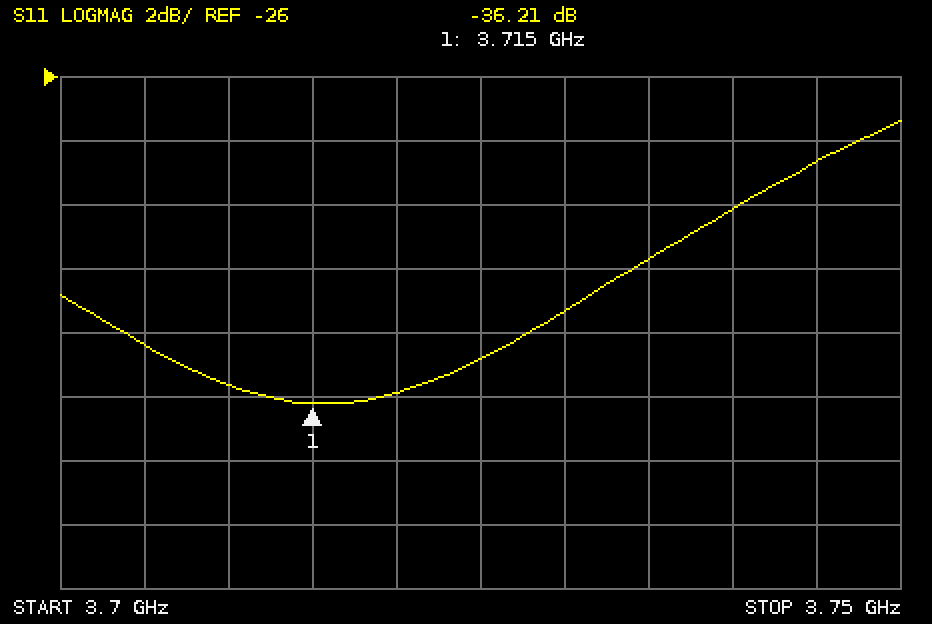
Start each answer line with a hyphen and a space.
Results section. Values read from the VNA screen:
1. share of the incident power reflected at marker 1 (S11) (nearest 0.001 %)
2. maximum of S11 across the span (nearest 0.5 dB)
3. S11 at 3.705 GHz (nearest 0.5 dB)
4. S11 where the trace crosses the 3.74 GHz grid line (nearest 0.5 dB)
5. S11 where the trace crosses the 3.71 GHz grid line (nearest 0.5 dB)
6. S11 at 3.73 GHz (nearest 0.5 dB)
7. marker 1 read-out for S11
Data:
- 0.024 %
- -27.5 dB
- -34.5 dB
- -30.0 dB
- -35.5 dB
- -33.5 dB
- -36.21 dB
